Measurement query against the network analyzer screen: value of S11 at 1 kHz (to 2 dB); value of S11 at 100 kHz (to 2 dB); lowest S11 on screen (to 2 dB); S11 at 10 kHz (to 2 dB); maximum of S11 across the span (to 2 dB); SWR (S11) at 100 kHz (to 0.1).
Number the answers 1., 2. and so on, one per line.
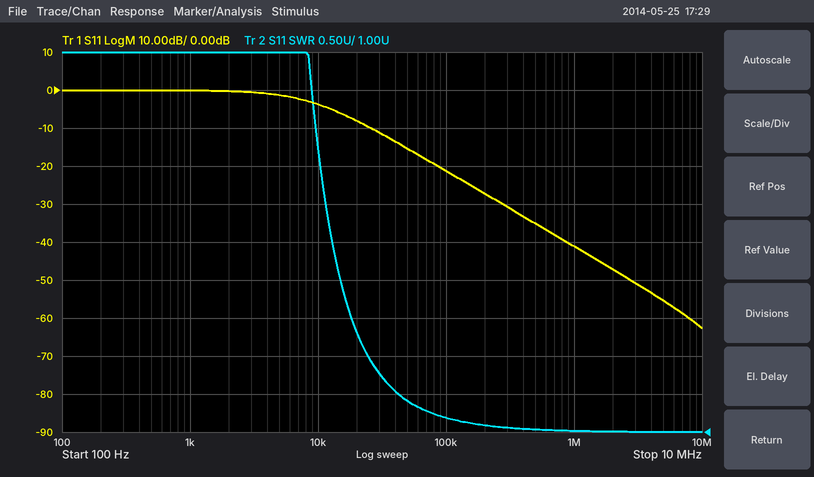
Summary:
1. 0 dB
2. -22 dB
3. -62 dB
4. -4 dB
5. 0 dB
6. 1.2
